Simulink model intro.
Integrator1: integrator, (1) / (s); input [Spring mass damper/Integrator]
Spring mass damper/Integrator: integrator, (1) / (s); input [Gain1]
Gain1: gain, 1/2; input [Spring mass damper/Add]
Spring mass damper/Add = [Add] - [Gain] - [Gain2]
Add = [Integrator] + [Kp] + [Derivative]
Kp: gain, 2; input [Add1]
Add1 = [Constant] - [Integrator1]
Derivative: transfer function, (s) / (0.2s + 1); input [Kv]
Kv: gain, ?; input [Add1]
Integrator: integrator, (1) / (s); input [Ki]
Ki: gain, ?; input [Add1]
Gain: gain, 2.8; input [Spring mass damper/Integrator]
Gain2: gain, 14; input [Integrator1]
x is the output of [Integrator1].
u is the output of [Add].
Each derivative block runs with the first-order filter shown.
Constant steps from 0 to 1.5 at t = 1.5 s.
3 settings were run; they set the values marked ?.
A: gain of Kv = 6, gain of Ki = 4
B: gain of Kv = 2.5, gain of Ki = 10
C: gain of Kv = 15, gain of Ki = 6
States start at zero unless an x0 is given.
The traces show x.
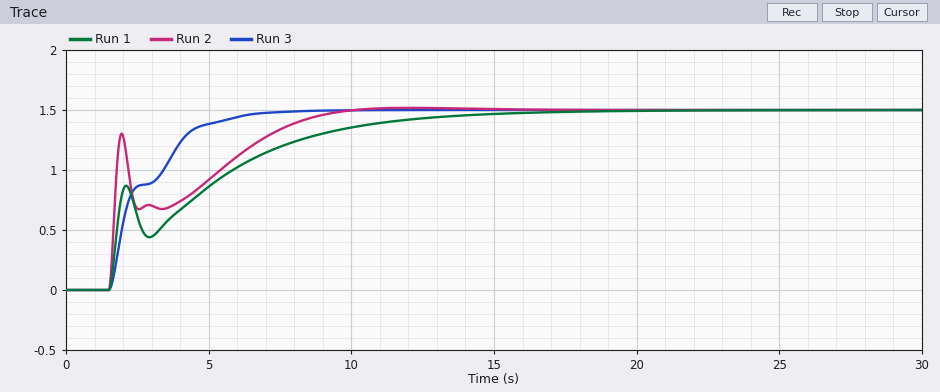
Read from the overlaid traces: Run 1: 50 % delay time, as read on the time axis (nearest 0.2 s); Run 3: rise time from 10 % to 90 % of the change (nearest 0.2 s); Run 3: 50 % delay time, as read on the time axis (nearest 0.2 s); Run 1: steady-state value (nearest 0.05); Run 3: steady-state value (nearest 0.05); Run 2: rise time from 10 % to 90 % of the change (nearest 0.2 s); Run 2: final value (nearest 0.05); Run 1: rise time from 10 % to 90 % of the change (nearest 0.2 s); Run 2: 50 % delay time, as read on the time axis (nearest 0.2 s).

2.0 s
2.8 s
2.2 s
1.50
1.50
6.0 s
1.50
8.2 s
1.8 s
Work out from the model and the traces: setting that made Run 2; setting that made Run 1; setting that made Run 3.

C
A
B
